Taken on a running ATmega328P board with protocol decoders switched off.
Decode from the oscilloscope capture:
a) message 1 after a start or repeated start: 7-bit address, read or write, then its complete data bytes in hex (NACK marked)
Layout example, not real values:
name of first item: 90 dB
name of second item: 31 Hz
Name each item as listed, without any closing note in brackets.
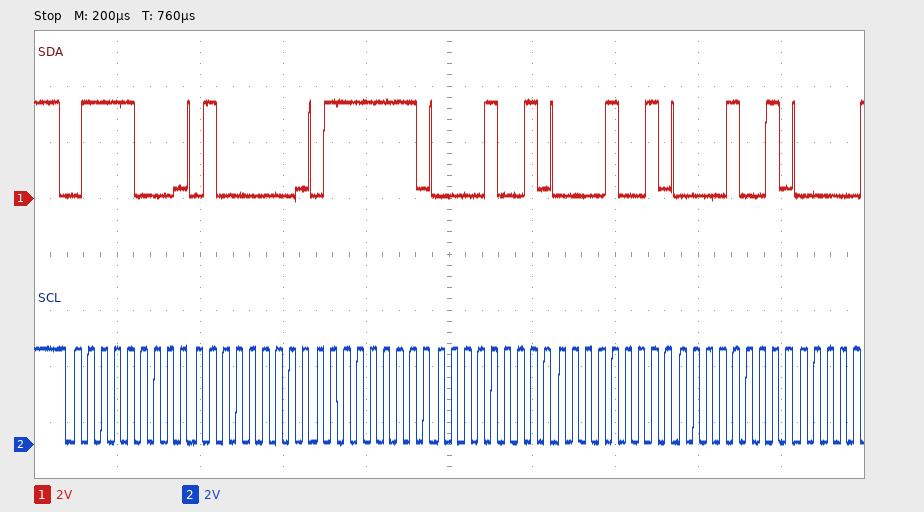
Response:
message 1 after a start or repeated start: 7-bit address, read or write, then its complete data bytes in hex: 0x3C write: 40 7F 09 09 09
